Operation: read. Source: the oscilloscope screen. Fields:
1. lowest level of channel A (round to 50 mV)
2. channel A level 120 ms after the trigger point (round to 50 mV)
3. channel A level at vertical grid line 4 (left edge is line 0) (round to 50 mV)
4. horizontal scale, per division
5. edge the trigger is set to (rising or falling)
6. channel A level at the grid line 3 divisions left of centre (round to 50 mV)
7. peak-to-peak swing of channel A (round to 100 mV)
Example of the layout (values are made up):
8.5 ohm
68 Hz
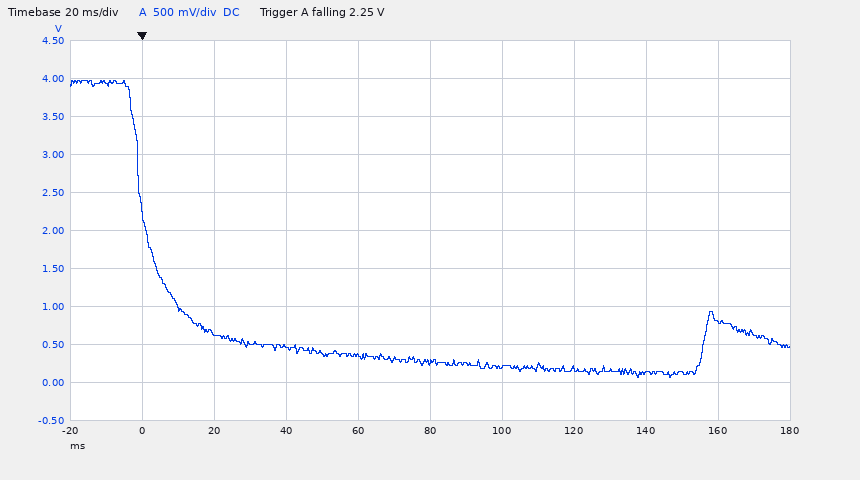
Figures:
50 mV
200 mV
350 mV
20 ms
falling
650 mV
3.90 V
